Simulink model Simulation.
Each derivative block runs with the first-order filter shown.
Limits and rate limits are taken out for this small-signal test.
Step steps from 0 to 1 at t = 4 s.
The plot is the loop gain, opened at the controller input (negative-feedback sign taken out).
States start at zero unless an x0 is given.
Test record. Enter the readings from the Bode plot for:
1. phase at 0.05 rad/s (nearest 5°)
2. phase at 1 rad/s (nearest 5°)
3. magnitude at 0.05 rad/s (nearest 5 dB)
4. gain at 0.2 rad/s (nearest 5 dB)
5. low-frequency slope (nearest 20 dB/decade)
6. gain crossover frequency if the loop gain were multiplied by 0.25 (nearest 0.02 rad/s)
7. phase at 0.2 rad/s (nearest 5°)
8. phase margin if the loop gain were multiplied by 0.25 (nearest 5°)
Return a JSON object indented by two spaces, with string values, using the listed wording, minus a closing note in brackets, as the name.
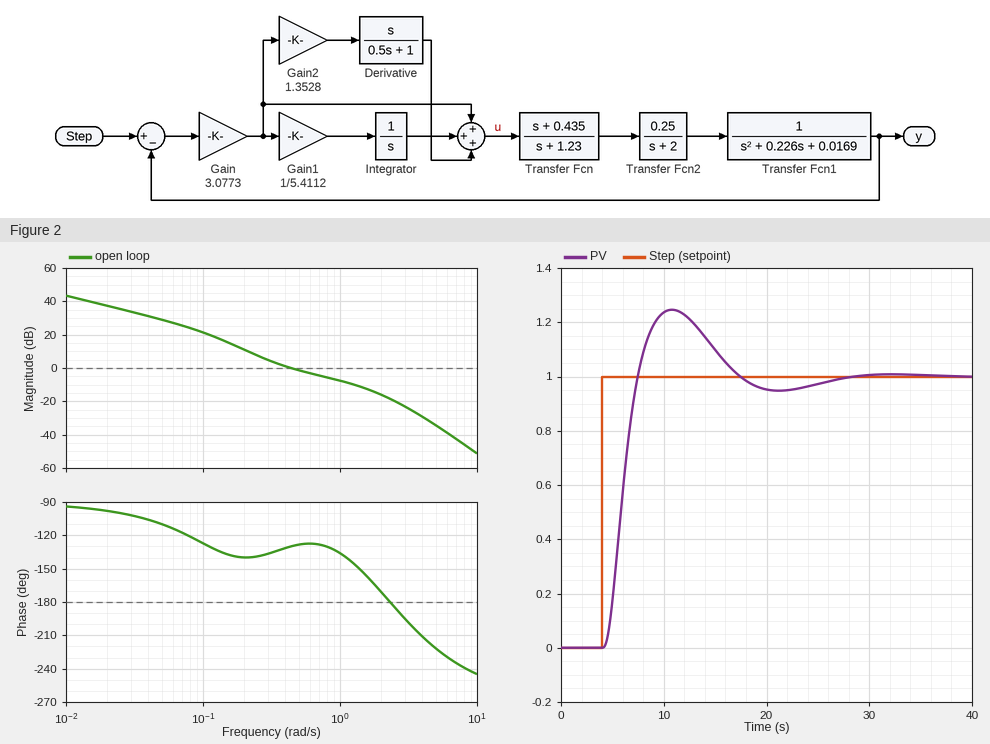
{
  "phase at 0.05 rad/s": "-110°",
  "phase at 1 rad/s": "-135°",
  "magnitude at 0.05 rad/s": "30 dB",
  "gain at 0.2 rad/s": "10 dB",
  "low-frequency slope": "-20 dB/decade",
  "gain crossover frequency if the loop gain were multiplied by 0.25": "0.18 rad/s",
  "phase at 0.2 rad/s": "-140°",
  "phase margin if the loop gain were multiplied by 0.25": "40°"
}
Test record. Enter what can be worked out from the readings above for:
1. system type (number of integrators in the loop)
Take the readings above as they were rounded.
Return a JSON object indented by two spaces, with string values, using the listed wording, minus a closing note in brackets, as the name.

{
  "system type": "1"
}
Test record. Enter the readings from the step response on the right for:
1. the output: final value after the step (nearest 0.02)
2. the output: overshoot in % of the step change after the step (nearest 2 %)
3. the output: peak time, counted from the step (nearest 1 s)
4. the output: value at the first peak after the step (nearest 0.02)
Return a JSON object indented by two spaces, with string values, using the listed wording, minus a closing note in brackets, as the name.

{
  "the output: final value after the step": "1.00",
  "the output: overshoot in % of the step change after the step": "24 %",
  "the output: peak time, counted from the step": "7 s",
  "the output: value at the first peak after the step": "1.24"
}
